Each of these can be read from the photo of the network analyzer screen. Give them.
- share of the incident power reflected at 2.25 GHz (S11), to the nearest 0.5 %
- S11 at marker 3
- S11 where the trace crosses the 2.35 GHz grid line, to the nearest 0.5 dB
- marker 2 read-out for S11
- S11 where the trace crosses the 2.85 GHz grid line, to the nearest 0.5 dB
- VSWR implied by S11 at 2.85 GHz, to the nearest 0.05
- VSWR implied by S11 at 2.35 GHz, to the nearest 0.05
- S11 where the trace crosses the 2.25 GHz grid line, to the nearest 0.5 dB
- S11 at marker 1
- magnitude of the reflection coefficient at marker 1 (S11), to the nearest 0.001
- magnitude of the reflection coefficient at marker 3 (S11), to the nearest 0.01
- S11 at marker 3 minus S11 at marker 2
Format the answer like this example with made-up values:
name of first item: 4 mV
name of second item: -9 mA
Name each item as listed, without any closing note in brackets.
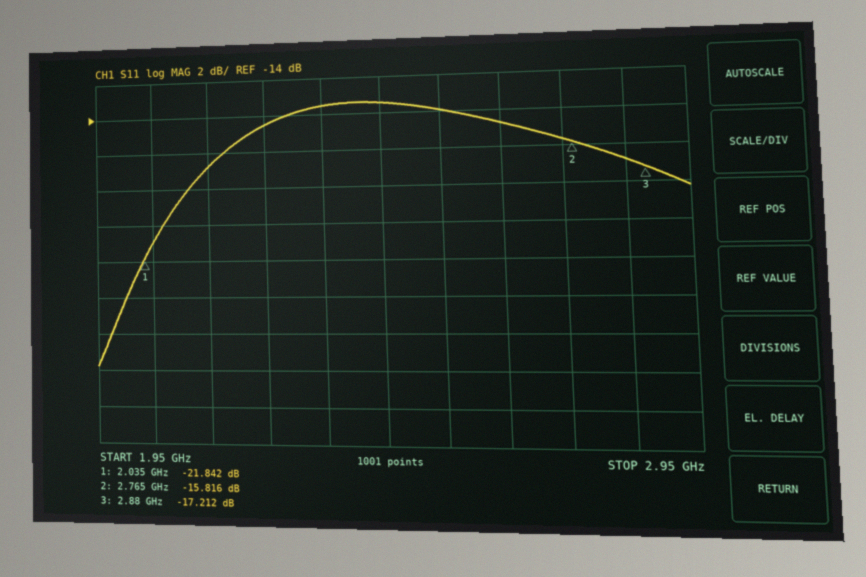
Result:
share of the incident power reflected at 2.25 GHz (S11), to the nearest 0.5 %: 3.5 %
S11 at marker 3: -17.212 dB
S11 where the trace crosses the 2.35 GHz grid line, to the nearest 0.5 dB: -13.5 dB
marker 2 read-out for S11: -15.816 dB
S11 where the trace crosses the 2.85 GHz grid line, to the nearest 0.5 dB: -17.0 dB
VSWR implied by S11 at 2.85 GHz, to the nearest 0.05: 1.35
VSWR implied by S11 at 2.35 GHz, to the nearest 0.05: 1.55
S11 where the trace crosses the 2.25 GHz grid line, to the nearest 0.5 dB: -14.5 dB
S11 at marker 1: -21.842 dB
magnitude of the reflection coefficient at marker 1 (S11), to the nearest 0.001: 0.081
magnitude of the reflection coefficient at marker 3 (S11), to the nearest 0.01: 0.14
S11 at marker 3 minus S11 at marker 2: -1.396 dB
